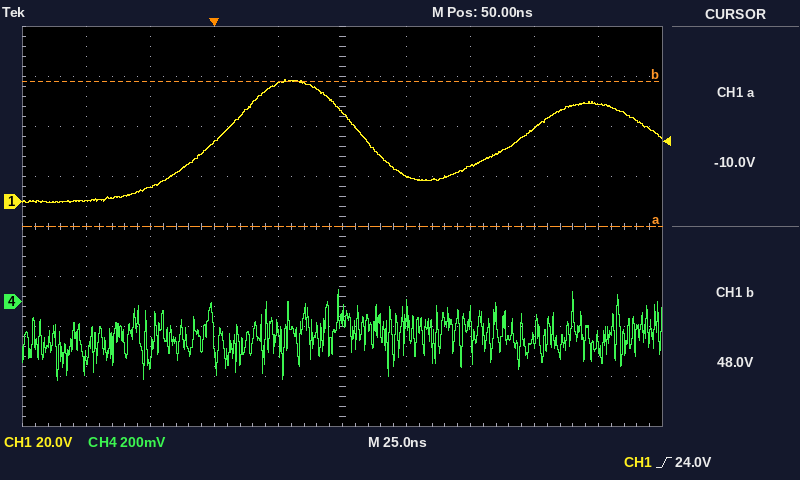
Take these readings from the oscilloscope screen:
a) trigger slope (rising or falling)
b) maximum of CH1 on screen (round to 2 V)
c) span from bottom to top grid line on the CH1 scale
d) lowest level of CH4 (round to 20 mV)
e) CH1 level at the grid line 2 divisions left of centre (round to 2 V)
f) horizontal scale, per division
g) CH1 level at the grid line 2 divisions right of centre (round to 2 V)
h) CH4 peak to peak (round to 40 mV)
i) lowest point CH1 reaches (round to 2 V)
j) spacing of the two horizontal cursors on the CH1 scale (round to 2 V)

rising
48 V
160 V
-320 mV
24 V
25 ns
14 V
360 mV
0 V
58 V
